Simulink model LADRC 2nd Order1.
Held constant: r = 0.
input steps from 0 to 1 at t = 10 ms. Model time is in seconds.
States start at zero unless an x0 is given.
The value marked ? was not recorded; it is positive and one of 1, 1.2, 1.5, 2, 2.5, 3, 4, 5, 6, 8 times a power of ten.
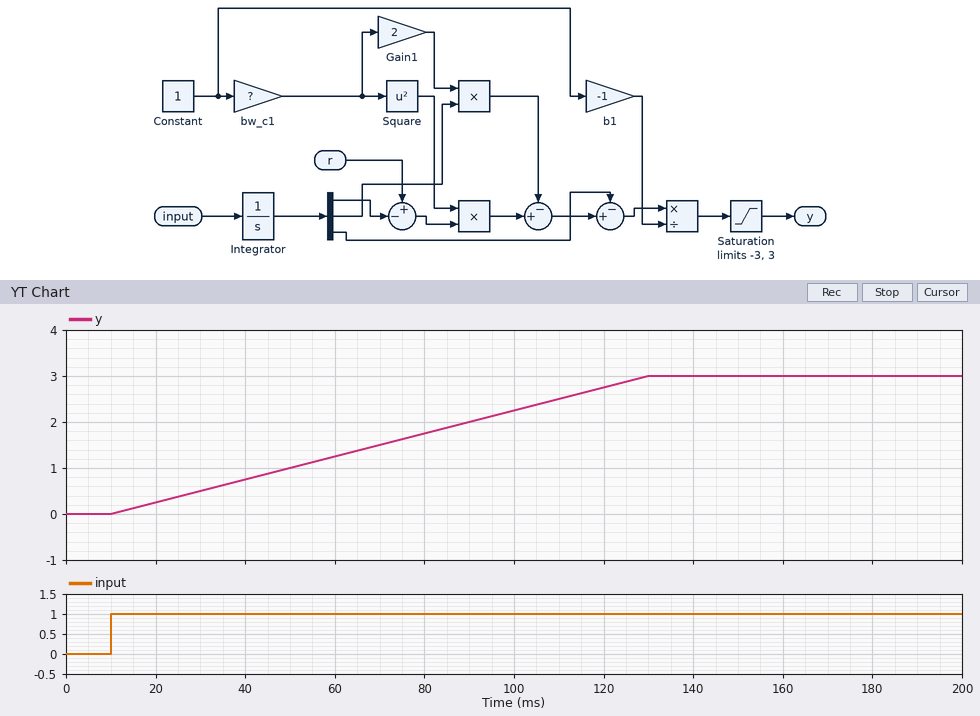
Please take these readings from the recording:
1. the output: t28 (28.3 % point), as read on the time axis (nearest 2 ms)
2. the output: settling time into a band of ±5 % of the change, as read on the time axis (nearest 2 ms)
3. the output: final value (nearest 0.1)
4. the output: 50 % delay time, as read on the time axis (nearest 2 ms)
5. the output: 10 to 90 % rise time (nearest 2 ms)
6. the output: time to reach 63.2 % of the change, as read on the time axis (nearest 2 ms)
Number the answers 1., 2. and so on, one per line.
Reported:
1. 44 ms
2. 124 ms
3. 3.0
4. 70 ms
5. 96 ms
6. 86 ms
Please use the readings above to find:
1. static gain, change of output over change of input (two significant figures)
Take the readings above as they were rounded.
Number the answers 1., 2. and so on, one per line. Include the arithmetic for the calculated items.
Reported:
1. (3 - 0) / (1 - 0) = 3.0
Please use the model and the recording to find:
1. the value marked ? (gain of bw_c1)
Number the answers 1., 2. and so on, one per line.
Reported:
1. 4
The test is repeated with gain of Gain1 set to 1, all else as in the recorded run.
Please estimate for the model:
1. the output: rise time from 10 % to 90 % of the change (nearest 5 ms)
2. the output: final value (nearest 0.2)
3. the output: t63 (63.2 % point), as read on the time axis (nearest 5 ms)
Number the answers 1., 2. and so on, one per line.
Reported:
1. 115 ms
2. 3.0
3. 100 ms
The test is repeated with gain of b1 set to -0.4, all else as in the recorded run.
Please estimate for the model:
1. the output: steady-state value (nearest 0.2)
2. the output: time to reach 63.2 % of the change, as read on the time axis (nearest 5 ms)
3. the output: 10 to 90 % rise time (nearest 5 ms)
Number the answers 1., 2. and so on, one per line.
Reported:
1. 3.0
2. 40 ms
3. 40 ms
